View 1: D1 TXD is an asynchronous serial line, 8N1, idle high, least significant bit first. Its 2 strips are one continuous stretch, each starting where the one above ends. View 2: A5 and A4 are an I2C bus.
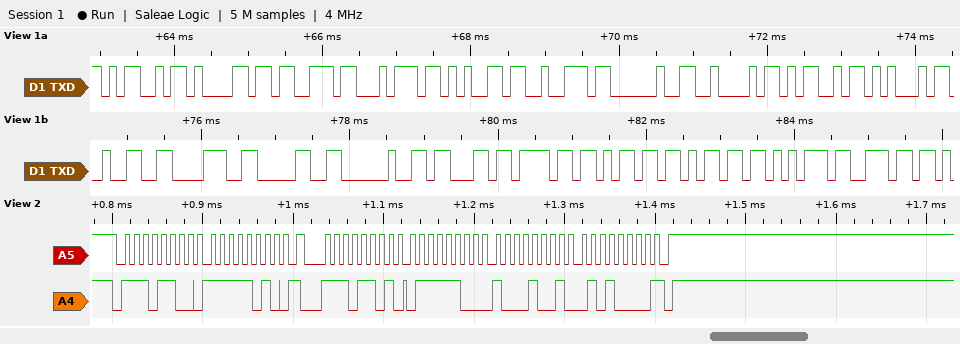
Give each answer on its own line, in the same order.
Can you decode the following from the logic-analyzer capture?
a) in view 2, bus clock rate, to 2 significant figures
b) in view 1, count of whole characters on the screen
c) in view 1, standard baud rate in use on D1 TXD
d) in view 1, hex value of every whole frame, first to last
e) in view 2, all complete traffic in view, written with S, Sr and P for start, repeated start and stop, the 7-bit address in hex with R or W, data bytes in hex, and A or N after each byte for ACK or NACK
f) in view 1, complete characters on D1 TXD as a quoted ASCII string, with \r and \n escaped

100 kHz
20
9600 baud
4D 61 73 74 65 72 20 42 4D 45 32 38 30 20 63 6F 6D 6D 75 6E
S 76W A FA A Sr 76R A 7C A 89 A 50 N P
"Master BME280 commun"
